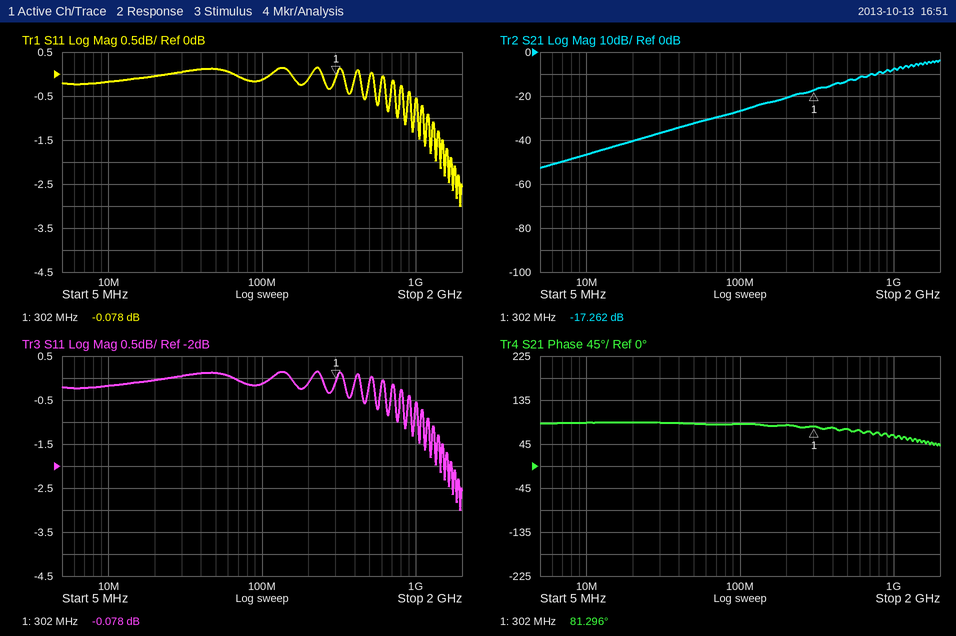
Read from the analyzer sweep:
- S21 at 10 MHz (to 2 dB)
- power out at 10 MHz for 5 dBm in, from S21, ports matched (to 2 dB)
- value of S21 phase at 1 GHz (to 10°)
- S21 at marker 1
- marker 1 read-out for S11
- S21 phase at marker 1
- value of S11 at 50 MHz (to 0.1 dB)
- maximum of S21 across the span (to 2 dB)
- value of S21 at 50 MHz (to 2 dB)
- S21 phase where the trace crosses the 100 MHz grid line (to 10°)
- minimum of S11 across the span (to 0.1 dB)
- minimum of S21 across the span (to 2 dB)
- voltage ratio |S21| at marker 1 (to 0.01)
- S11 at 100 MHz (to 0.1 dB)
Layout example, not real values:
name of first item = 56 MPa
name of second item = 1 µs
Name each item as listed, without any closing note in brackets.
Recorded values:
S21 at 10 MHz = -46 dB
power out at 10 MHz for 5 dBm in, from S21, ports matched = -42 dBm
value of S21 phase at 1 GHz = 60°
S21 at marker 1 = -17.262 dB
marker 1 read-out for S11 = -0.078 dB
S21 phase at marker 1 = 81.296°
value of S11 at 50 MHz = 0.1 dB
maximum of S21 across the span = -4 dB
value of S21 at 50 MHz = -32 dB
S21 phase where the trace crosses the 100 MHz grid line = 90°
minimum of S11 across the span = -3.0 dB
minimum of S21 across the span = -52 dB
voltage ratio |S21| at marker 1 = 0.14
S11 at 100 MHz = -0.1 dB
